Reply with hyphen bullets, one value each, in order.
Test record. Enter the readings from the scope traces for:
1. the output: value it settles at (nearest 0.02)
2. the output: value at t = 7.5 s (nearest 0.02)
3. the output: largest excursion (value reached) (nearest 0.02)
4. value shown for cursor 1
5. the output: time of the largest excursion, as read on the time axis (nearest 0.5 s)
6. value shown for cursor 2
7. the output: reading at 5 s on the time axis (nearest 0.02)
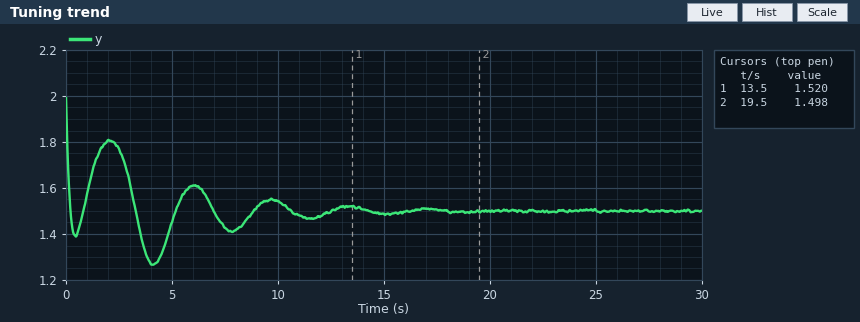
- 1.50
- 1.42
- 1.26
- 1.520
- 4.0 s
- 1.498
- 1.46
